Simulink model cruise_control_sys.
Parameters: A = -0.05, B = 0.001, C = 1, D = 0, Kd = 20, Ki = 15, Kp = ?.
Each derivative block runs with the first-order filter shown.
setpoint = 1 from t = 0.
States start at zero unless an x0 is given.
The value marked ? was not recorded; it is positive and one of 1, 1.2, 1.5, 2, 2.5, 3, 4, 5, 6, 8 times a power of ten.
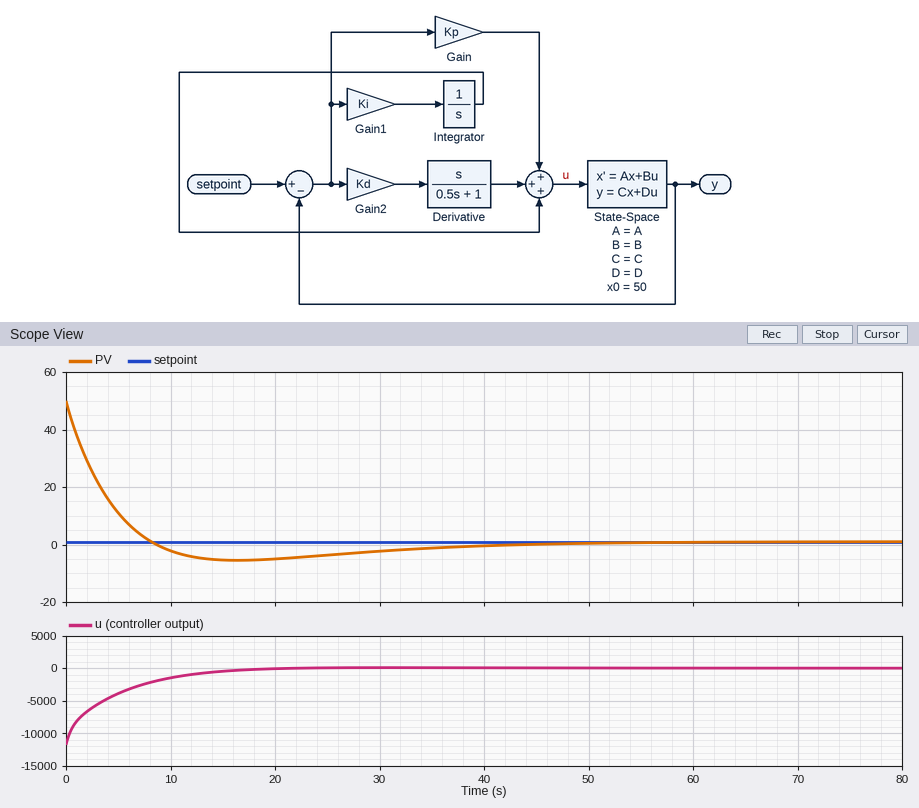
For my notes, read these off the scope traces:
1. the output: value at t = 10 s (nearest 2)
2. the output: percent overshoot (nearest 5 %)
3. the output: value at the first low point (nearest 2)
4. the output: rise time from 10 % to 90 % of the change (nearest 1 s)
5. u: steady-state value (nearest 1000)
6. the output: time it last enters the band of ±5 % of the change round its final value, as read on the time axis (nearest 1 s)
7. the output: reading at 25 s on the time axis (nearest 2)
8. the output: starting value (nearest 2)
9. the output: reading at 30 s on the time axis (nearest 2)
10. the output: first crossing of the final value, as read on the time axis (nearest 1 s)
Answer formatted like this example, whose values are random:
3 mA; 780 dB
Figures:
-2; 15 %; -6; 6 s; 0; 34 s; -4; 50; -2; 8 s
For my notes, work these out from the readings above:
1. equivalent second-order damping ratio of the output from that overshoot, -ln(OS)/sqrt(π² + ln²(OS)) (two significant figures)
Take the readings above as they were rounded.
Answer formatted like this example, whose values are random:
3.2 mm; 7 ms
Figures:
0.52
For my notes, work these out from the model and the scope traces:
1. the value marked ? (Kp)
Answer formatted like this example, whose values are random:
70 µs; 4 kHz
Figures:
200
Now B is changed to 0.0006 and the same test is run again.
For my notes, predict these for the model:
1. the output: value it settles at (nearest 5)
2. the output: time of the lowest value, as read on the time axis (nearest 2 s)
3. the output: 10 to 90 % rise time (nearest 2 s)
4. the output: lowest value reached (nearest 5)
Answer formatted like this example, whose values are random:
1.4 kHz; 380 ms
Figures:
0; 22 s; 8 s; -5
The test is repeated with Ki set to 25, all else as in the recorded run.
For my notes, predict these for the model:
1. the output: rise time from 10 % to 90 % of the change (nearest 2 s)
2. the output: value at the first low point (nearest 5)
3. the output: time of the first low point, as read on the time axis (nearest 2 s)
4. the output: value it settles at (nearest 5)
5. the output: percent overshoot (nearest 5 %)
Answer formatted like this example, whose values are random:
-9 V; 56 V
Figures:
6 s; -10; 14 s; 0; 20 %
